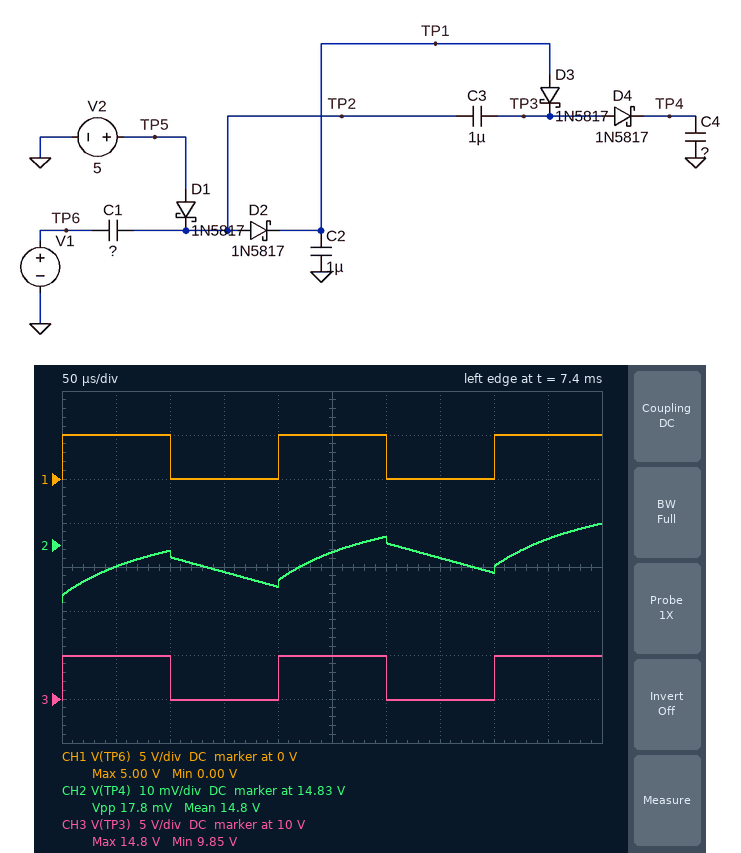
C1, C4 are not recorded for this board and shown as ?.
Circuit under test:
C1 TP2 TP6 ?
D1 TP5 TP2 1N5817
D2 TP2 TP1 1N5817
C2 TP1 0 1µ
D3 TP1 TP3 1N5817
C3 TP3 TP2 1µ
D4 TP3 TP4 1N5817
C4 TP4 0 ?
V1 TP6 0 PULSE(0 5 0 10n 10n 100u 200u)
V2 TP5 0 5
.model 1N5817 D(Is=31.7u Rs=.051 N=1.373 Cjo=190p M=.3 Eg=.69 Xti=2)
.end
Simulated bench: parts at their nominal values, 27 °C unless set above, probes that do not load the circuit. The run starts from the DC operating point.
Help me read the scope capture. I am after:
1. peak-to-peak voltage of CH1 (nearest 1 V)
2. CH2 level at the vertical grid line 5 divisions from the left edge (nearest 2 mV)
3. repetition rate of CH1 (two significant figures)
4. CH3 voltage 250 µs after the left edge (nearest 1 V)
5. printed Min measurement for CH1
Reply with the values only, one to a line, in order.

5 V
14.828 V
5.0 kHz
15 V
0.00 V
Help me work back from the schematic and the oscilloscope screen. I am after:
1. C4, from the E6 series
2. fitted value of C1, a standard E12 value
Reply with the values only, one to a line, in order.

470 nF
2.7 µF
